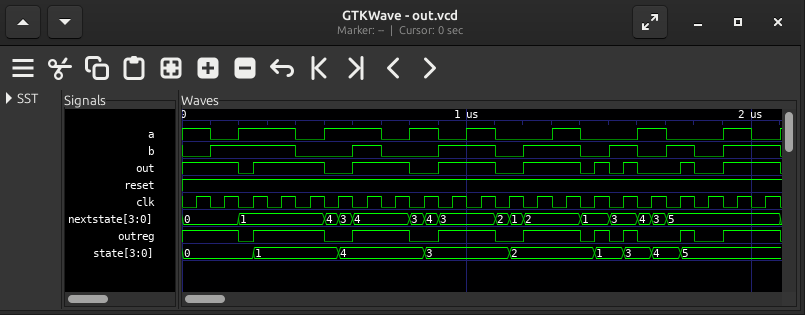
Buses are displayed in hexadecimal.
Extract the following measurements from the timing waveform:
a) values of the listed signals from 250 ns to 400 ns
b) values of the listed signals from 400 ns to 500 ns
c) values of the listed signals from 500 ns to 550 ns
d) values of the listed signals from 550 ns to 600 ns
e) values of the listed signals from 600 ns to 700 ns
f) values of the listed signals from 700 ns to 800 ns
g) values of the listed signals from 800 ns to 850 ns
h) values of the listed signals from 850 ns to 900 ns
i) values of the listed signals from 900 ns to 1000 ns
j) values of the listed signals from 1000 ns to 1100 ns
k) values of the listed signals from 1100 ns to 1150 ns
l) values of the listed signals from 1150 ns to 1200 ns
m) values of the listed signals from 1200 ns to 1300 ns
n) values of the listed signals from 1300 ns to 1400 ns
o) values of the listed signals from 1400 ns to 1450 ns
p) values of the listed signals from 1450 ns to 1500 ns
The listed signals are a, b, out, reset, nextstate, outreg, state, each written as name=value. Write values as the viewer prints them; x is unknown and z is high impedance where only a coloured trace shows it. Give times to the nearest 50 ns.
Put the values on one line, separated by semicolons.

a=1, b=1, out=1, reset=1, nextstate=1, outreg=1, state=1; a=0, b=0, out=1, reset=1, nextstate=1, outreg=1, state=1; a=1, b=0, out=0, reset=1, nextstate=4, outreg=0, state=1; a=1, b=0, out=0, reset=1, nextstate=3, outreg=0, state=4; a=1, b=1, out=1, reset=1, nextstate=4, outreg=1, state=4; a=0, b=0, out=1, reset=1, nextstate=4, outreg=1, state=4; a=1, b=0, out=0, reset=1, nextstate=3, outreg=0, state=4; a=1, b=0, out=0, reset=1, nextstate=4, outreg=0, state=3; a=0, b=1, out=1, reset=1, nextstate=3, outreg=1, state=3; a=1, b=1, out=1, reset=1, nextstate=3, outreg=1, state=3; a=0, b=0, out=0, reset=1, nextstate=2, outreg=0, state=3; a=0, b=0, out=0, reset=1, nextstate=1, outreg=0, state=2; a=0, b=1, out=1, reset=1, nextstate=2, outreg=1, state=2; a=1, b=1, out=1, reset=1, nextstate=2, outreg=1, state=2; a=0, b=0, out=0, reset=1, nextstate=1, outreg=0, state=2; a=0, b=0, out=1, reset=1, nextstate=1, outreg=1, state=1
